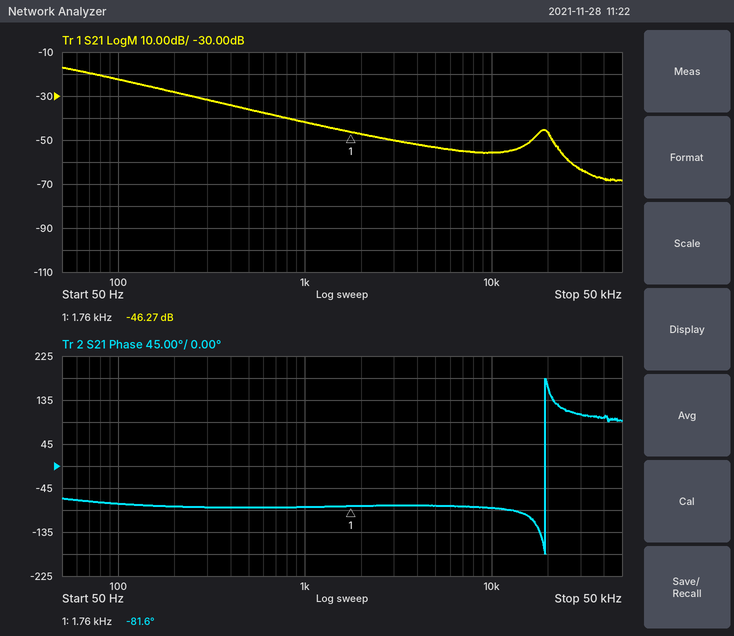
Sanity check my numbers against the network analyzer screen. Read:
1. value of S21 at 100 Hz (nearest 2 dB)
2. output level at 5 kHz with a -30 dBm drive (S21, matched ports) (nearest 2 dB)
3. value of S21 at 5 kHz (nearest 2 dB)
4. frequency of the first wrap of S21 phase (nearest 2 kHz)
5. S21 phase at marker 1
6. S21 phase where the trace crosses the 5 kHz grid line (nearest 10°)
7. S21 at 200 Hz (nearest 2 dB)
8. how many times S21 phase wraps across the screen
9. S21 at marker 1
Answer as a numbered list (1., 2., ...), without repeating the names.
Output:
1. -22 dB
2. -84 dBm
3. -54 dB
4. 20 kHz
5. -81.6°
6. -80°
7. -28 dB
8. 1
9. -46.27 dB
